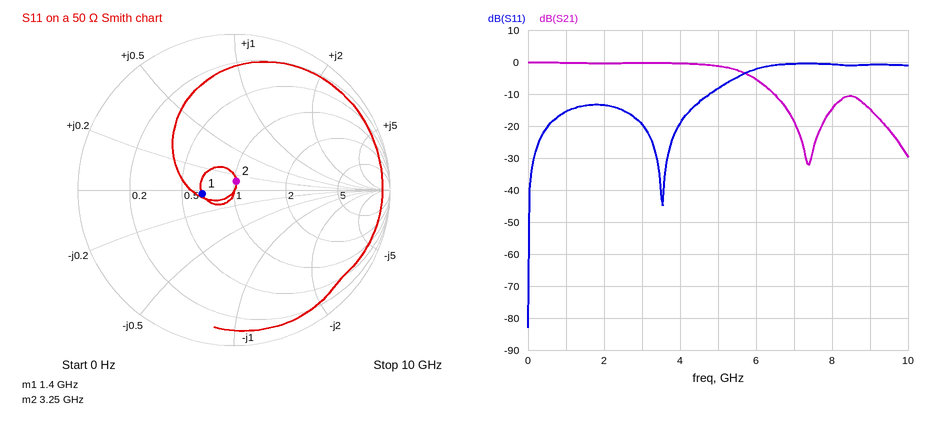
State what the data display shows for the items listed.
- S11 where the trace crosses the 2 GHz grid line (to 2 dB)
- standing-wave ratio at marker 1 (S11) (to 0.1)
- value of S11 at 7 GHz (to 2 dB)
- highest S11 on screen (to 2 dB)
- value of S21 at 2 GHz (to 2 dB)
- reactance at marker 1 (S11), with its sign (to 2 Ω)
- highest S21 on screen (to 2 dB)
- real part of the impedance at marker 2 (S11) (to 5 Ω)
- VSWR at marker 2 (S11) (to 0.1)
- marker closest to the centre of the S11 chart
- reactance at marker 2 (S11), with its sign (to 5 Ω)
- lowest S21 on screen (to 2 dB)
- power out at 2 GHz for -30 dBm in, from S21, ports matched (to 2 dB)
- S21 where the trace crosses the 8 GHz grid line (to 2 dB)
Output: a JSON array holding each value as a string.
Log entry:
["-14 dB", "1.5", "0 dB", "0 dB", "0 dB", "-2 Ω", "0 dB", "50 Ω", "1.1", "marker 2", "+5 Ω", "-32 dB", "-30 dBm", "-14 dB"]
